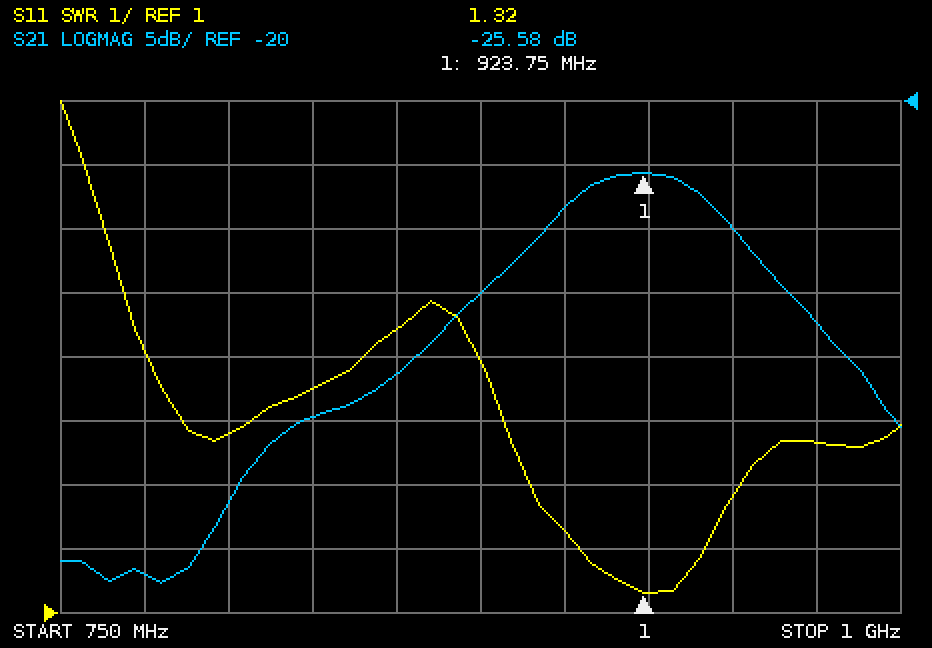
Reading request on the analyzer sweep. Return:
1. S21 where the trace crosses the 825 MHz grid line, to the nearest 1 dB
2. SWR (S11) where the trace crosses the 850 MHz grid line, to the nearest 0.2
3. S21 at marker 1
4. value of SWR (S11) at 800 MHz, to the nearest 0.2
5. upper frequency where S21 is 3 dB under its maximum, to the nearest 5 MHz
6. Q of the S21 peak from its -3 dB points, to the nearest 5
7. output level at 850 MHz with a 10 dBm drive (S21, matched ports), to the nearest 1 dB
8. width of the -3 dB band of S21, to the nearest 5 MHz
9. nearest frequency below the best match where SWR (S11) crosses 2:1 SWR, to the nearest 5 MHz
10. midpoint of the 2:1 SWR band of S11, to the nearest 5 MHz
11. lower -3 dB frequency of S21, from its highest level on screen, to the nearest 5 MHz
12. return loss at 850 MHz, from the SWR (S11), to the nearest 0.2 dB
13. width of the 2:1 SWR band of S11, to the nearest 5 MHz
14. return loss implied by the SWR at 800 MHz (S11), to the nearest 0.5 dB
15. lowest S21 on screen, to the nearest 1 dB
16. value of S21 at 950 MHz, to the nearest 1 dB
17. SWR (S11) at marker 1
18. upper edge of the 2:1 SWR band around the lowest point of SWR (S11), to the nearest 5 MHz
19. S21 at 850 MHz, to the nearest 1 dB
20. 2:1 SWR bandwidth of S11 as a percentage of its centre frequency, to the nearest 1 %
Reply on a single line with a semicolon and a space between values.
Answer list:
-45 dB; 5.4; -25.58 dB; 3.8; 945 MHz; 20; -31 dBm; 45 MHz; 905 MHz; 925 MHz; 900 MHz; 3.2 dB; 35 MHz; 4.5 dB; -58 dB; -30 dB; 1.32; 940 MHz; -41 dB; 4 %
